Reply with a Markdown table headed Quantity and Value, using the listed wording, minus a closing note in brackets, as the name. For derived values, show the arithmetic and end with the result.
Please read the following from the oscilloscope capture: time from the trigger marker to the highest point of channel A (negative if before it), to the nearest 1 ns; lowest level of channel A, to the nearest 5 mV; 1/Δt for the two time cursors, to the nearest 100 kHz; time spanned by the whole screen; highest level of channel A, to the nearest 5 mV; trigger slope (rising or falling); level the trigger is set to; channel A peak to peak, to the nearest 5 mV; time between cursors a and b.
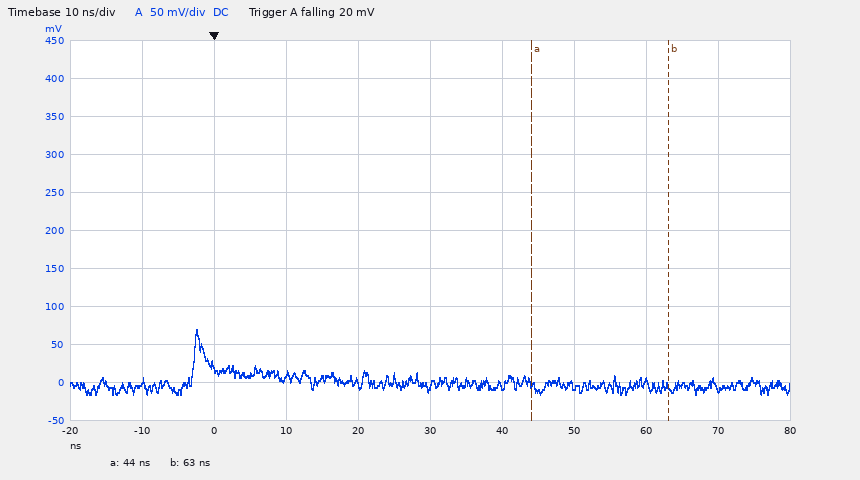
| Quantity | Value |
|---|---|
| time from the trigger marker to the highest point of channel A (negative if before it), to the nearest 1 ns | -2 ns |
| lowest level of channel A, to the nearest 5 mV | -15 mV |
| 1/Δt for the two time cursors, to the nearest 100 kHz | 1 / 19 ns ≈ 52.6 MHz |
| time spanned by the whole screen | 100 ns |
| highest level of channel A, to the nearest 5 mV | 70 mV |
| trigger slope | falling |
| level the trigger is set to | 20 mV |
| channel A peak to peak, to the nearest 5 mV | 70 mV − (-15 mV) = 85 mV |
| time between cursors a and b | 63 ns − (44 ns) = 19 ns |
